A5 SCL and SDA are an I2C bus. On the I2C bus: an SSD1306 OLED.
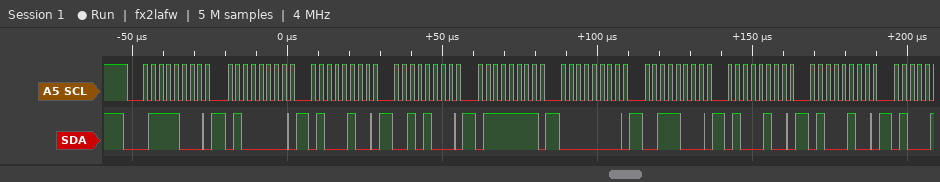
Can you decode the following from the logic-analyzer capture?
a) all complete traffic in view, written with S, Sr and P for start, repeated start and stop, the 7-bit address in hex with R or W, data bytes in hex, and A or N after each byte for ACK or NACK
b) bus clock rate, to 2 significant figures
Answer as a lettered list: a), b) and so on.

a) S 3CW A 40 A 44 A 28 A 7F A 00 A 38 A 44 A 44 A
b) 400 kHz
